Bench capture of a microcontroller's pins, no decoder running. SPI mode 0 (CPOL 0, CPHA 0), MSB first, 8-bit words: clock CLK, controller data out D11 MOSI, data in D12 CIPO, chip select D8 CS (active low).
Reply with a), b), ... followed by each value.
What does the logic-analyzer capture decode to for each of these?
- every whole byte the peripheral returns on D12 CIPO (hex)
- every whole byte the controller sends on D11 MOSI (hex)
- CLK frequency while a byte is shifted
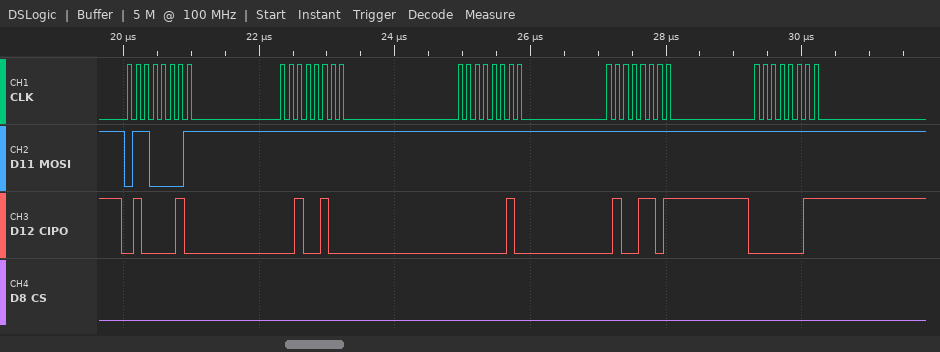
a) 42 24 02 4D 03
b) 61 FF FF FF FF
c) 8 MHz
